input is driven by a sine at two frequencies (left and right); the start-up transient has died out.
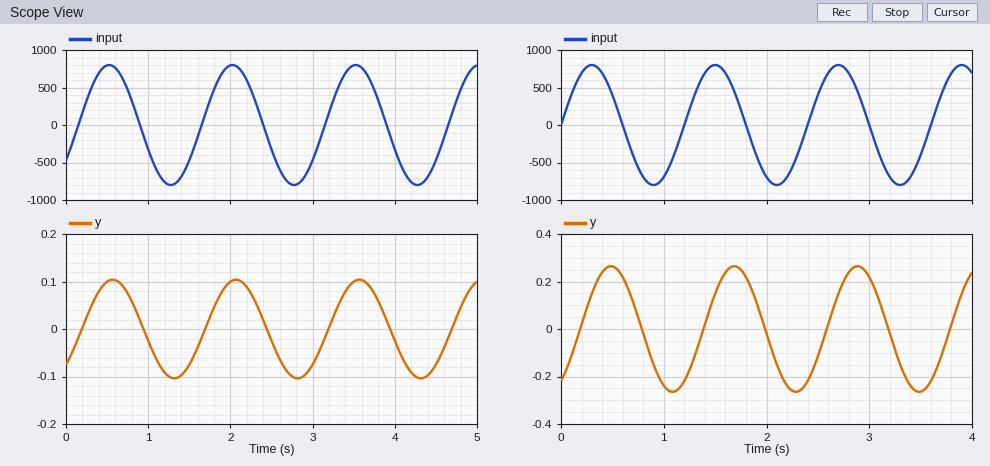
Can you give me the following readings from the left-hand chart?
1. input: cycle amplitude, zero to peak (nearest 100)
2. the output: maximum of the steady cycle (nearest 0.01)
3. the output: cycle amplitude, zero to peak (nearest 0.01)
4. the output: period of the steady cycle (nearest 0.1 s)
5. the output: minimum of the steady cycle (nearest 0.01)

800
0.10
0.10
1.5 s
-0.10
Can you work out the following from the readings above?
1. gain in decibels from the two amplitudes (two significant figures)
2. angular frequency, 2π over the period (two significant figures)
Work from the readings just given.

-78 dB
4.2 rad/s
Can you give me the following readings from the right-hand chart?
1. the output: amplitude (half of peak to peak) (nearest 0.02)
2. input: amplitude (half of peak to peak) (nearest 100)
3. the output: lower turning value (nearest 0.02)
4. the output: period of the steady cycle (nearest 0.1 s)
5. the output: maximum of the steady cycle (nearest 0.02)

0.26
800
-0.26
1.2 s
0.26
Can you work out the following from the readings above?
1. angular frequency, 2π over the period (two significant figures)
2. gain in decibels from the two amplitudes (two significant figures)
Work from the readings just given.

5.2 rad/s
-70 dB
